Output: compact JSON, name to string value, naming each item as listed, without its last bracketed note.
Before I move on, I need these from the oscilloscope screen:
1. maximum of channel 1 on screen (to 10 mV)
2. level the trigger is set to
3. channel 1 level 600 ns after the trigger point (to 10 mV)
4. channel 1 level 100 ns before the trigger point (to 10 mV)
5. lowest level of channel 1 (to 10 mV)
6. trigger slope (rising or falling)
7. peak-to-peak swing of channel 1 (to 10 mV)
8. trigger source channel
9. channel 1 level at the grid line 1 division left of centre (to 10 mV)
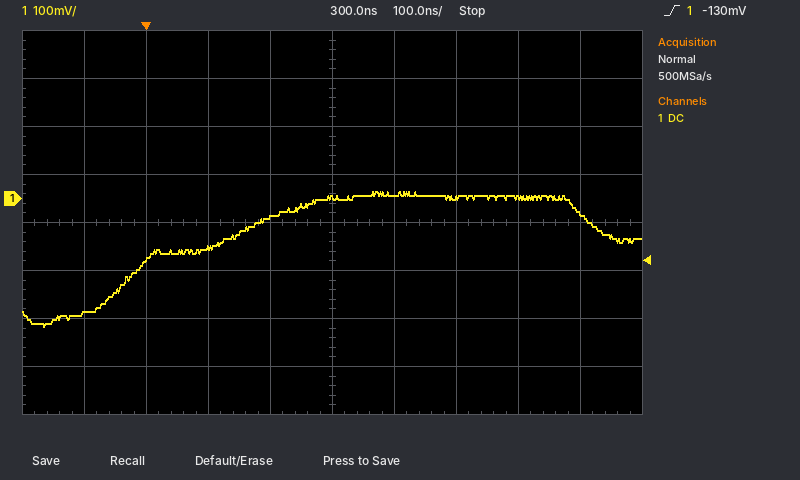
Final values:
{"maximum of channel 1 on screen": "10 mV", "level the trigger is set to": "-130 mV", "channel 1 level 600 ns after the trigger point": "0 mV", "channel 1 level 100 ns before the trigger point": "-240 mV", "lowest level of channel 1": "-270 mV", "trigger slope": "rising", "peak-to-peak swing of channel 1": "280 mV", "trigger source channel": "channel 1", "channel 1 level at the grid line 1 division left of centre": "-40 mV"}
